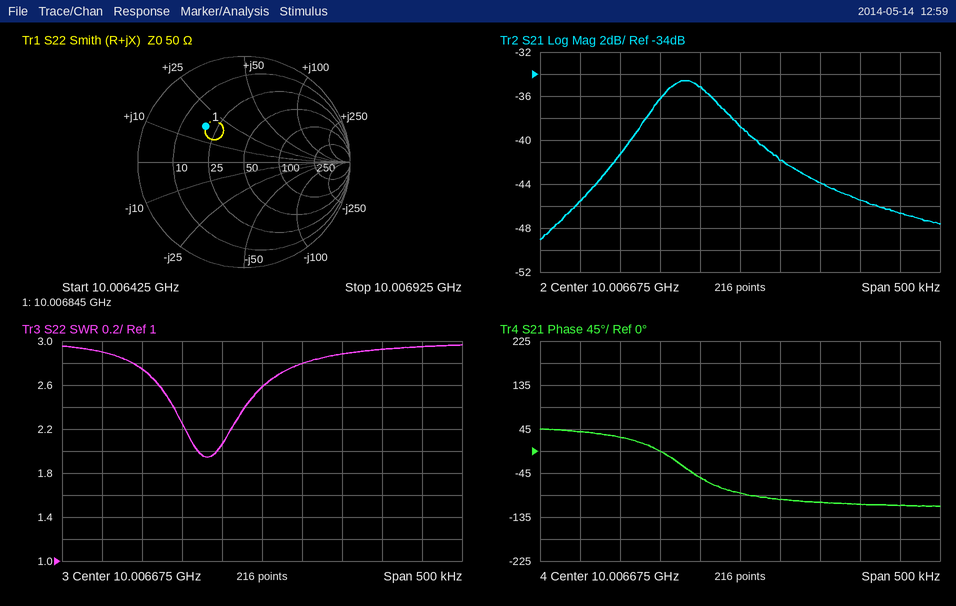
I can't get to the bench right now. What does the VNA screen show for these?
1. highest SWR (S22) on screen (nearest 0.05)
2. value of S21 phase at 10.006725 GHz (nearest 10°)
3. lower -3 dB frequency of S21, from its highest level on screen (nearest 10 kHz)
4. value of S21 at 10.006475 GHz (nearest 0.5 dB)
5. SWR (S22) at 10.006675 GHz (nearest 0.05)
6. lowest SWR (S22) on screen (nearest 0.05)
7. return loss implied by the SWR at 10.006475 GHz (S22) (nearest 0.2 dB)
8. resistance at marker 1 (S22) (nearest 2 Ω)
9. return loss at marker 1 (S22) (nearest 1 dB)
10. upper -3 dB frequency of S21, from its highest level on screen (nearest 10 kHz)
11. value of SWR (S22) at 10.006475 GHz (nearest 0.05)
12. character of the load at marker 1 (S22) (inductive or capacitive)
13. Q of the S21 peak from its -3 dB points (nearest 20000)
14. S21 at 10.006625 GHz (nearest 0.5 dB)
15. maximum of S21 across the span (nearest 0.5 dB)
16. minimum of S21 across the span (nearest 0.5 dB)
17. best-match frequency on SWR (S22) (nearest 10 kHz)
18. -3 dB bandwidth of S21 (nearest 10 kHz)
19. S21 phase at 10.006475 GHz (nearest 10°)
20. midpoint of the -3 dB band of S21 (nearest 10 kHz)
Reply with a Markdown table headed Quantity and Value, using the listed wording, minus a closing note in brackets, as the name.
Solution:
| Quantity | Value |
|---|---|
| highest SWR (S22) on screen | 2.95 |
| value of S21 phase at 10.006725 GHz | -100° |
| lower -3 dB frequency of S21, from its highest level on screen | 10.00656 GHz |
| value of S21 at 10.006475 GHz | -45.5 dB |
| SWR (S22) at 10.006675 GHz | 2.60 |
| lowest SWR (S22) on screen | 1.95 |
| return loss implied by the SWR at 10.006475 GHz (S22) | 6.2 dB |
| resistance at marker 1 (S22) | 20 Ω |
| return loss at marker 1 (S22) | 6 dB |
| upper -3 dB frequency of S21, from its highest level on screen | 10.00666 GHz |
| value of SWR (S22) at 10.006475 GHz | 2.90 |
| character of the load at marker 1 (S22) | inductive |
| Q of the S21 peak from its -3 dB points | 100000 |
| S21 at 10.006625 GHz | -35.0 dB |
| maximum of S21 across the span | -34.5 dB |
| minimum of S21 across the span | -49.0 dB |
| best-match frequency on SWR (S22) | 10.00661 GHz |
| -3 dB bandwidth of S21 | 100 kHz |
| S21 phase at 10.006475 GHz | 40° |
| midpoint of the -3 dB band of S21 | 10.00661 GHz |
